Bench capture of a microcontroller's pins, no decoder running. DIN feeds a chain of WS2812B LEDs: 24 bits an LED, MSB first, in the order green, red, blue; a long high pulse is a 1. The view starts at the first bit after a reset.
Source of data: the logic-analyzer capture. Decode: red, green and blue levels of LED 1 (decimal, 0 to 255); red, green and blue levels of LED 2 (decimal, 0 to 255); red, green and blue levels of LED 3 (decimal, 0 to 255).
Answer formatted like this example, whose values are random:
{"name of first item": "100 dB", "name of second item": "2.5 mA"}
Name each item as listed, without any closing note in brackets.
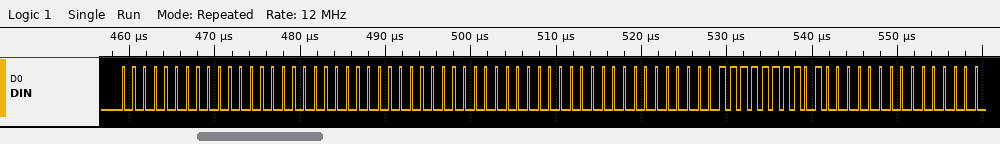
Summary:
{"red, green and blue levels of LED 1": "0, 0, 0", "red, green and blue levels of LED 2": "0, 0, 0", "red, green and blue levels of LED 3": "255, 0, 64"}
